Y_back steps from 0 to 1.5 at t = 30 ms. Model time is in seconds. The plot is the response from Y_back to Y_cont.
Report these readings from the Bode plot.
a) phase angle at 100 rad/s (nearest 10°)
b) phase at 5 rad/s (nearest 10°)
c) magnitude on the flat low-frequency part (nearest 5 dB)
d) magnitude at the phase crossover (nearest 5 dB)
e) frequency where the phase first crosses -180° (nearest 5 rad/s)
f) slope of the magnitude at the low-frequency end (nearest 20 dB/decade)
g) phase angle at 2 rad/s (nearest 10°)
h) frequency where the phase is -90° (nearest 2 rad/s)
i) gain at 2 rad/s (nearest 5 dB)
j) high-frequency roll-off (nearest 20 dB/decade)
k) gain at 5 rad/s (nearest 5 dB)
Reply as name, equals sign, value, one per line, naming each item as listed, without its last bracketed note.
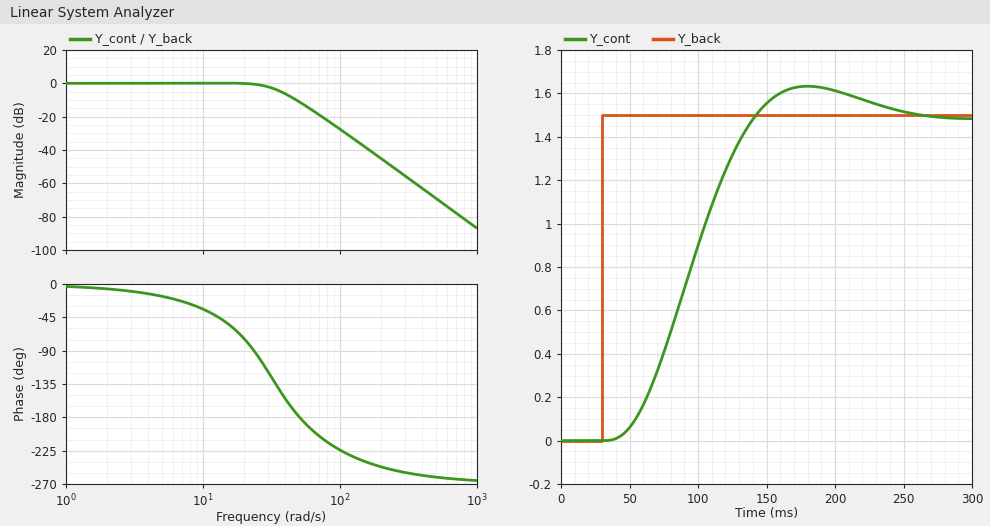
phase angle at 100 rad/s = -220°
phase at 5 rad/s = -20°
magnitude on the flat low-frequency part = 0 dB
magnitude at the phase crossover = -10 dB
frequency where the phase first crosses -180° = 50 rad/s
slope of the magnitude at the low-frequency end = 0 dB/decade
phase angle at 2 rad/s = -10°
frequency where the phase is -90° = 24 rad/s
gain at 2 rad/s = 0 dB
high-frequency roll-off = -60 dB/decade
gain at 5 rad/s = 0 dB
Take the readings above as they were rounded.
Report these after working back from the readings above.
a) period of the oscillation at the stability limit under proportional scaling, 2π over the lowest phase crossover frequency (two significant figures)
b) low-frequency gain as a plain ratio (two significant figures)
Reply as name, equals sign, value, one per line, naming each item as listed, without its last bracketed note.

period of the oscillation at the stability limit under proportional scaling, 2π over the lowest phase crossover frequency = 0.13 s
low-frequency gain as a plain ratio = 1.0
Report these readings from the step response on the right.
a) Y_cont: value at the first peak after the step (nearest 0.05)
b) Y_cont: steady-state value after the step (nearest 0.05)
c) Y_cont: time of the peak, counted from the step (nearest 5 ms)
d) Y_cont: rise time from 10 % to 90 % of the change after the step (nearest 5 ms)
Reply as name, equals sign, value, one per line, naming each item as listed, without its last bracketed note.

Y_cont: value at the first peak after the step = 1.65
Y_cont: steady-state value after the step = 1.50
Y_cont: time of the peak, counted from the step = 150 ms
Y_cont: rise time from 10 % to 90 % of the change after the step = 70 ms
